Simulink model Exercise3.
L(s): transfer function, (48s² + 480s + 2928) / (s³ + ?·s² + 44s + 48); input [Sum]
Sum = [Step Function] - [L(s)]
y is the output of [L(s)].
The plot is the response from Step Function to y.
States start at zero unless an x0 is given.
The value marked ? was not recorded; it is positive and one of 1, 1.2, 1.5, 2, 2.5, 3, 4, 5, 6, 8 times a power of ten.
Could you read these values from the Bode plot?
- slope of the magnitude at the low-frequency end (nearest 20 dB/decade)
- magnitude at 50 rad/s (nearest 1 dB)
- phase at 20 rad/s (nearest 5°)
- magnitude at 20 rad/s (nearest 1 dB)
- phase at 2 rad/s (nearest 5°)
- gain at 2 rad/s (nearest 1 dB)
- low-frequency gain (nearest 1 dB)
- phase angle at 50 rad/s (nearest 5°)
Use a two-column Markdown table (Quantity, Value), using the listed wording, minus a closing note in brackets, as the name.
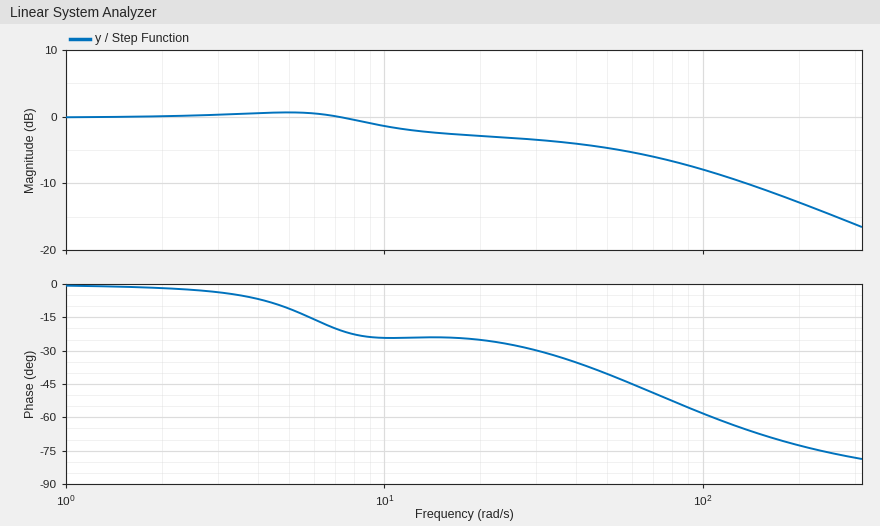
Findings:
| Quantity | Value |
|---|---|
| slope of the magnitude at the low-frequency end | 0 dB/decade |
| magnitude at 50 rad/s | -5 dB |
| phase at 20 rad/s | -25° |
| magnitude at 20 rad/s | -3 dB |
| phase at 2 rad/s | 0° |
| gain at 2 rad/s | 0 dB |
| low-frequency gain | 0 dB |
| phase angle at 50 rad/s | -40° |
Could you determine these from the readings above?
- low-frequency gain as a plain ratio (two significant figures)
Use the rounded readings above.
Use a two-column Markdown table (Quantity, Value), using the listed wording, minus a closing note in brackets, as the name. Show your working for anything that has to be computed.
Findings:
| Quantity | Value |
|---|---|
| low-frequency gain as a plain ratio | 10^(0 / 20) = 1.0 |
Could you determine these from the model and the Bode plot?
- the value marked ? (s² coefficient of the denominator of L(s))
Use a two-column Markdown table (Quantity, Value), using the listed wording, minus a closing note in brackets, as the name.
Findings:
| Quantity | Value |
|---|---|
| the value marked ? (s² coefficient of the denominator of L(s)) | 25 |
